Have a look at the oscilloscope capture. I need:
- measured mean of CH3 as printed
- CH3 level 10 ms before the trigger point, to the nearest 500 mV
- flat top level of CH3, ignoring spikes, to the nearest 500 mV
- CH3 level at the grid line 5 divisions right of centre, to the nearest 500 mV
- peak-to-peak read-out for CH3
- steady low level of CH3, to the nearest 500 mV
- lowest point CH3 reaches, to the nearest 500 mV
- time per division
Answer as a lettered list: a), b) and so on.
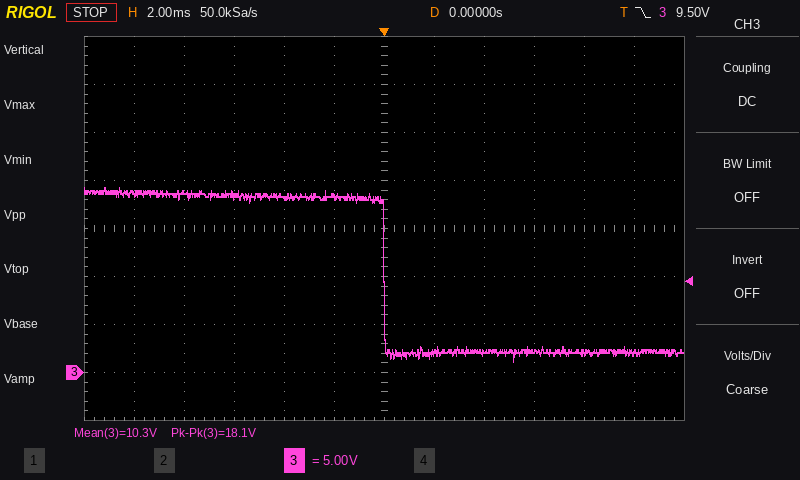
a) 10.3 V
b) 18.5 V
c) 18.5 V
d) 2.0 V
e) 18.1 V
f) 2.0 V
g) 1.0 V
h) 2 ms
